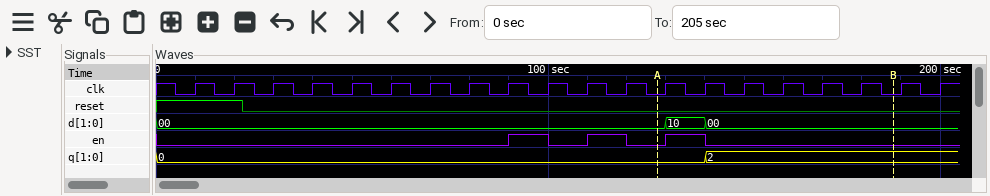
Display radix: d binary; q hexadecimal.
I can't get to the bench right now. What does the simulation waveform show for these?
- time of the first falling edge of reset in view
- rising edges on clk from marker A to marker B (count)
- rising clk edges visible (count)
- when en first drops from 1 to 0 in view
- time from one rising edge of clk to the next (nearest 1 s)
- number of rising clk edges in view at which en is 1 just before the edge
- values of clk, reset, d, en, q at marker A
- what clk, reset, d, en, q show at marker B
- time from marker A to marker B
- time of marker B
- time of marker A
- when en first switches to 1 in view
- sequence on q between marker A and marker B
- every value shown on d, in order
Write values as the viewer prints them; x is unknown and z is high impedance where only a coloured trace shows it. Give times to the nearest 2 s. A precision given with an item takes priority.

22 s
6
20
100 s
10 s
3
clk=0, reset=0, d=00, en=0, q=0
clk=0, reset=0, d=00, en=0, q=2
60 s
188 s
128 s
90 s
0, 2
00, 10, 00
